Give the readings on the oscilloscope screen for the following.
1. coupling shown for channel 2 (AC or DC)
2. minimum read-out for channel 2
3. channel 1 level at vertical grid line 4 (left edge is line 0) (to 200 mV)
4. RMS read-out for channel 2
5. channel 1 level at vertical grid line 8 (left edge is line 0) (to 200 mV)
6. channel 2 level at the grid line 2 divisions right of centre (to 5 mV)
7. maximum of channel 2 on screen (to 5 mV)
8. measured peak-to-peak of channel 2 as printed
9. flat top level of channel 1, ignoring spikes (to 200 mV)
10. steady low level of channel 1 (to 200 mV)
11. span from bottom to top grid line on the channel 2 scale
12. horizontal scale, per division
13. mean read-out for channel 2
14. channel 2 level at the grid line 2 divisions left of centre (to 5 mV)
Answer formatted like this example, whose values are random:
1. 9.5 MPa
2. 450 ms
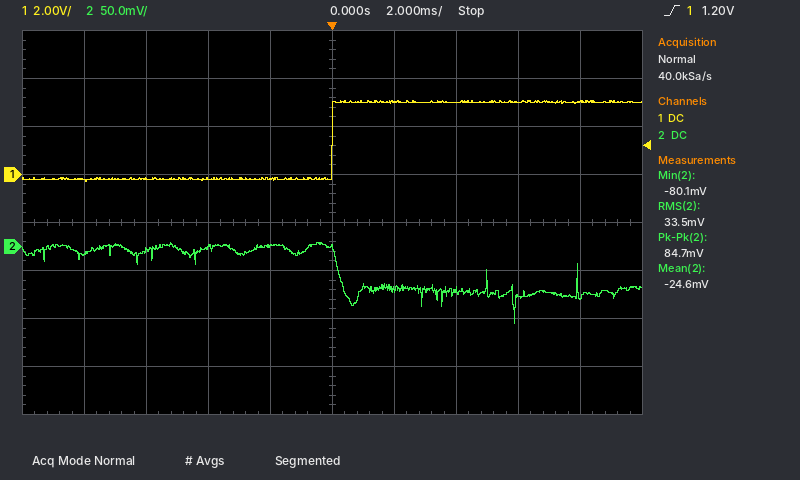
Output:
1. DC
2. -80.1 mV
3. -200 mV
4. 33.5 mV
5. 3.0 V
6. -45 mV
7. 5 mV
8. 84.7 mV
9. 3.0 V
10. -200 mV
11. 400 mV
12. 2 ms
13. -24.6 mV
14. 0 mV
